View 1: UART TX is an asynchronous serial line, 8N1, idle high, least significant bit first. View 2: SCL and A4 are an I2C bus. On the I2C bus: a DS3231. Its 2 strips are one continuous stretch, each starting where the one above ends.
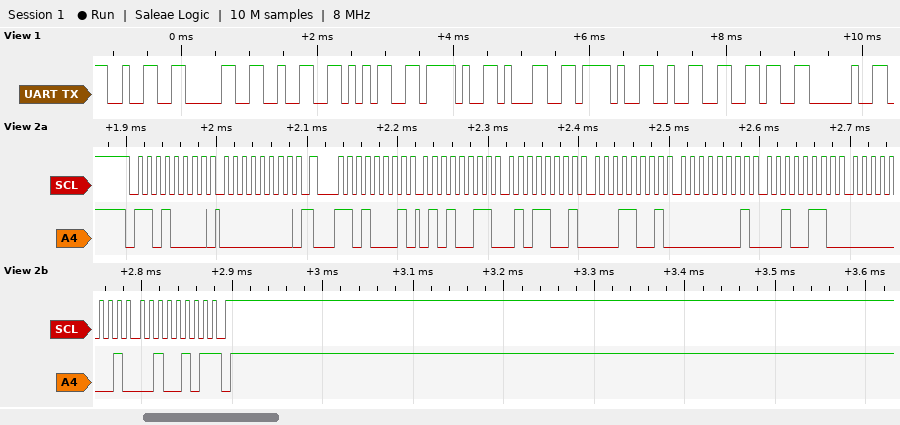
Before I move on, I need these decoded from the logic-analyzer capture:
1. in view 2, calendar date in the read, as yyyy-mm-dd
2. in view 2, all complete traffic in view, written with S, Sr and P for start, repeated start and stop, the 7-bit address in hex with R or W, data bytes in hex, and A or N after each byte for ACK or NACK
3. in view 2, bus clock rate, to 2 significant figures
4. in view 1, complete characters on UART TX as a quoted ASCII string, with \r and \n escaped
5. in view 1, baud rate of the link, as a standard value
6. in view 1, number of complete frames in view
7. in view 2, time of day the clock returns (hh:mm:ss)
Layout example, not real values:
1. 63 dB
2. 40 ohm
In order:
1. 2025-01-26
2. S 68W A 00 A Sr 68R A 53 A 59 A 19 A 01 A 26 A 01 A 25 N P
3. 100 kHz
4. "2025/1/26 "
5. 9600 baud
6. 10
7. 19:59:53
